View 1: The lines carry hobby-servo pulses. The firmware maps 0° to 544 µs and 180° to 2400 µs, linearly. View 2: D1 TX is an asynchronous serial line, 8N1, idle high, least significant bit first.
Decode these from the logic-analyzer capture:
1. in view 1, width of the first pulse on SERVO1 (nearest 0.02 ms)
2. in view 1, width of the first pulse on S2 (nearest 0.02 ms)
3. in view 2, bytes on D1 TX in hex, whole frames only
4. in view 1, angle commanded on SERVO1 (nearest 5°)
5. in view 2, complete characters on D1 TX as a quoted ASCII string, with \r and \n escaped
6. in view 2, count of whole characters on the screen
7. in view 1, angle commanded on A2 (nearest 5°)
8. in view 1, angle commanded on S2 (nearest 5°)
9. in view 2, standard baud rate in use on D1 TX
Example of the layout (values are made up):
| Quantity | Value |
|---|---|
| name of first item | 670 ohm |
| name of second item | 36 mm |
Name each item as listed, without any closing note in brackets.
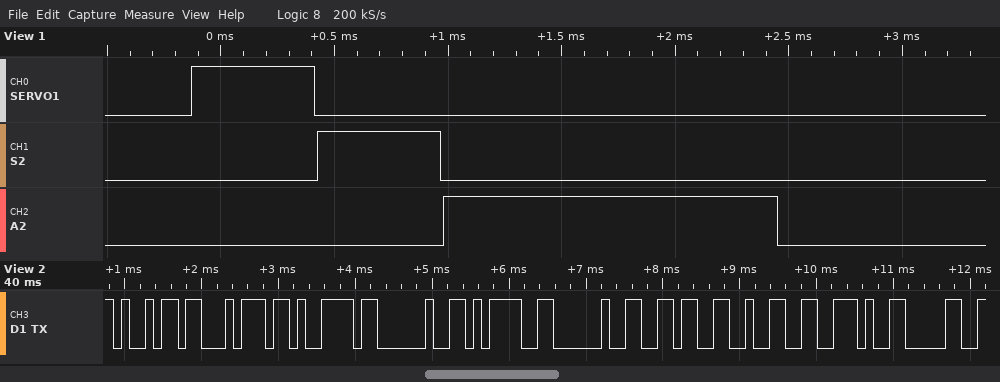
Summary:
| Quantity | Value |
|---|---|
| in view 1, width of the first pulse on SERVO1 | 0.54 ms |
| in view 1, width of the first pulse on S2 | 0.54 ms |
| in view 2, bytes on D1 TX in hex, whole frames only | 69 74 79 20 3D 20 36 32 2E 30 |
| in view 1, angle commanded on SERVO1 | 0° |
| in view 2, complete characters on D1 TX as a quoted ASCII string, with \r and \n escaped | "ity = 62.0" |
| in view 2, count of whole characters on the screen | 10 |
| in view 1, angle commanded on A2 | 90° |
| in view 1, angle commanded on S2 | 0° |
| in view 2, standard baud rate in use on D1 TX | 9600 baud |
